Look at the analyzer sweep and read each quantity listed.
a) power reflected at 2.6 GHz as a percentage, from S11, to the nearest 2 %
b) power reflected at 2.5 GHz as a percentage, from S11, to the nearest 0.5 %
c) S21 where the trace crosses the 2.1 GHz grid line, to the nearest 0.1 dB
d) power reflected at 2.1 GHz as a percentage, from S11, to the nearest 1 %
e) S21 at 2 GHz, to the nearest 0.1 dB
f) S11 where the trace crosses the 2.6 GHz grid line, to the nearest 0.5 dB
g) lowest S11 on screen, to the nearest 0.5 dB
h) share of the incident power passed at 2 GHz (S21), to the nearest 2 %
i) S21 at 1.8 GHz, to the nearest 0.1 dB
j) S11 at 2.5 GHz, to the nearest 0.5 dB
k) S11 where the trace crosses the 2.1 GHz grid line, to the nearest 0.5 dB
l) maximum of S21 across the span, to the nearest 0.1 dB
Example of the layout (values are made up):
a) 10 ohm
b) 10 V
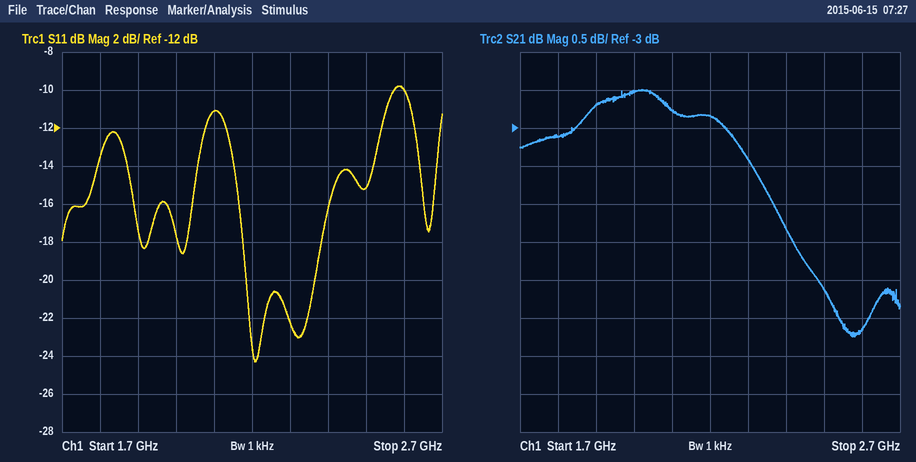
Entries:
a) 10 %
b) 3.0 %
c) -2.8 dB
d) 8 %
e) -2.5 dB
f) -10.0 dB
g) -24.5 dB
h) 56 %
i) -3.1 dB
j) -15.0 dB
k) -11.0 dB
l) -2.5 dB
